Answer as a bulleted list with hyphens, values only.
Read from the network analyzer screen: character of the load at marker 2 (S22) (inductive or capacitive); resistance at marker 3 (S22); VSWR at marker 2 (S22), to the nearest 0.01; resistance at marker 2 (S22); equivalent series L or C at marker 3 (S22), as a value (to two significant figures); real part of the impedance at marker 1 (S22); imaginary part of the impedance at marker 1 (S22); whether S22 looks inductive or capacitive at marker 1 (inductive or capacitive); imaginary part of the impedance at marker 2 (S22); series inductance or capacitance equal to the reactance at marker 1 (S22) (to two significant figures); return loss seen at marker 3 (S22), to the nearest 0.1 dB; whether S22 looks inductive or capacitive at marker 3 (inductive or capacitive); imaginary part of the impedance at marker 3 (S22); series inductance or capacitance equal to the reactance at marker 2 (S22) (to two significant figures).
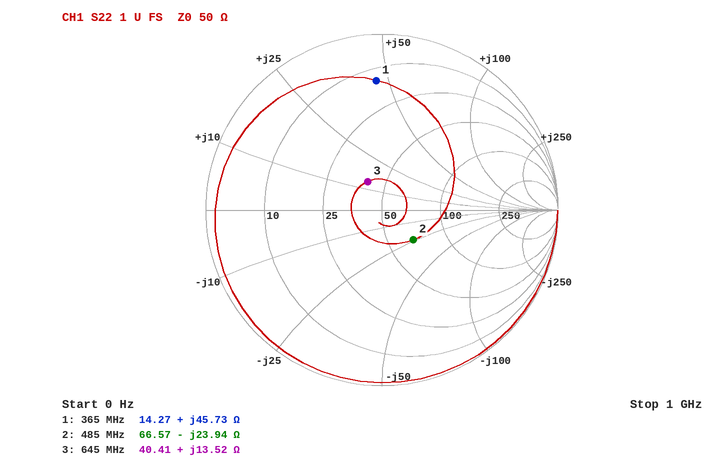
- capacitive
- 40.41 Ω
- 1.65
- 66.57 Ω
- 3.3 nH
- 14.27 Ω
- +45.73 Ω
- inductive
- -23.94 Ω
- 20 nH
- 14.8 dB
- inductive
- +13.52 Ω
- 14 pF
